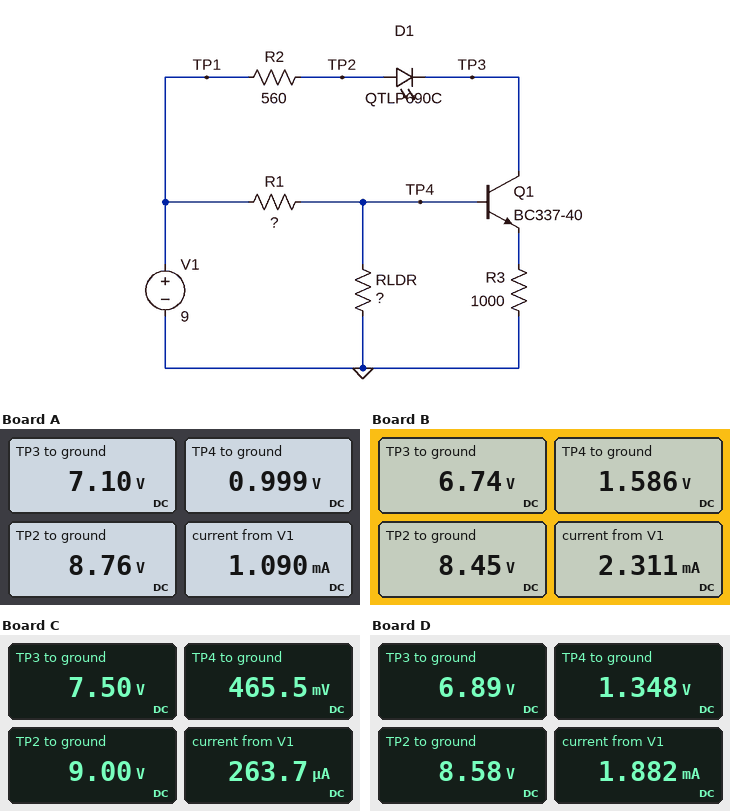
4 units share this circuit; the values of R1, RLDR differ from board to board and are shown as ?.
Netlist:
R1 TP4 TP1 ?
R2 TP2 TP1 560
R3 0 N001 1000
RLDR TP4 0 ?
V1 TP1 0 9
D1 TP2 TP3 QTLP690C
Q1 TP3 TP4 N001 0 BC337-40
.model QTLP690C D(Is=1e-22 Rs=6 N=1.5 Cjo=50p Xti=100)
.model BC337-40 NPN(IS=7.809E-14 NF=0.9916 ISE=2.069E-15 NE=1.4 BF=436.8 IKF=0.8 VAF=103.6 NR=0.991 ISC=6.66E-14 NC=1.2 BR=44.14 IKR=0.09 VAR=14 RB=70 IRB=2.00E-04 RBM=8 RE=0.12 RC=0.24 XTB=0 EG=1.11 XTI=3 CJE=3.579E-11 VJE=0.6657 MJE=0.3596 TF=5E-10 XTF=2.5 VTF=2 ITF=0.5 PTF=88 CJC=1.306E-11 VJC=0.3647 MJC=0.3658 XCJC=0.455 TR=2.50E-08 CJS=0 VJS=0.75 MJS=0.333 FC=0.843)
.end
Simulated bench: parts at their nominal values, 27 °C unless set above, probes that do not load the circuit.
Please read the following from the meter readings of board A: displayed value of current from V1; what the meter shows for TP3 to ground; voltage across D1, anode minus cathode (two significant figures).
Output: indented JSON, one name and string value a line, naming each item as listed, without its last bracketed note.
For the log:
{
  "displayed value of current from V1": "1.090 mA",
  "what the meter shows for TP3 to ground": "7.10 V",
  "voltage across D1, anode minus cathode": "1.7 V"
}
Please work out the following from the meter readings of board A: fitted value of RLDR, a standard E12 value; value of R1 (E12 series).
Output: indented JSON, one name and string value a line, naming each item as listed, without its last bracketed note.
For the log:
{
  "fitted value of RLDR, a standard E12 value": "1.5 kΩ",
  "value of R1": "12 kΩ"
}
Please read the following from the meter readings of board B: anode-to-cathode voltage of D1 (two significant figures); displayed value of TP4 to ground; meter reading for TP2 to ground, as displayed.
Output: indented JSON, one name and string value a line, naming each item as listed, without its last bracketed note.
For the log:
{
  "anode-to-cathode voltage of D1": "1.7 V",
  "displayed value of TP4 to ground": "1.586 V",
  "meter reading for TP2 to ground, as displayed": "8.45 V"
}
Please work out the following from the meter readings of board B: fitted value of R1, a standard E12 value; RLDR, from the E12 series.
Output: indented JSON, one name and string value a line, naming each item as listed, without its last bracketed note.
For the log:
{
  "fitted value of R1, a standard E12 value": "5.6 kΩ",
  "RLDR, from the E12 series": "1.2 kΩ"
}
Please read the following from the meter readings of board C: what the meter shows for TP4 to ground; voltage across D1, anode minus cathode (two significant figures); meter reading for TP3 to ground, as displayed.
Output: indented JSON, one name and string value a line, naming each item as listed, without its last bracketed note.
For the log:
{
  "what the meter shows for TP4 to ground": "465.5 mV",
  "voltage across D1, anode minus cathode": "1.5 V",
  "meter reading for TP3 to ground, as displayed": "7.50 V"
}
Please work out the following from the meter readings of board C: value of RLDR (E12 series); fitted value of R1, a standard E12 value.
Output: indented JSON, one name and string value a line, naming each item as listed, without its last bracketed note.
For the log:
{
  "value of RLDR": "1.8 kΩ",
  "fitted value of R1, a standard E12 value": "33 kΩ"
}
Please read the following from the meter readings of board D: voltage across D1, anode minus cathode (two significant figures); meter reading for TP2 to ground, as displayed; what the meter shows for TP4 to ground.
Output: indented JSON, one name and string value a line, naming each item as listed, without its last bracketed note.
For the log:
{
  "voltage across D1, anode minus cathode": "1.7 V",
  "meter reading for TP2 to ground, as displayed": "8.58 V",
  "what the meter shows for TP4 to ground": "1.348 V"
}
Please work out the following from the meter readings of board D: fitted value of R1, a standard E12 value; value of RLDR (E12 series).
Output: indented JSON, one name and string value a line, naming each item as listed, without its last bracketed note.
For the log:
{
  "fitted value of R1, a standard E12 value": "6.8 kΩ",
  "value of RLDR": "1.2 kΩ"
}
